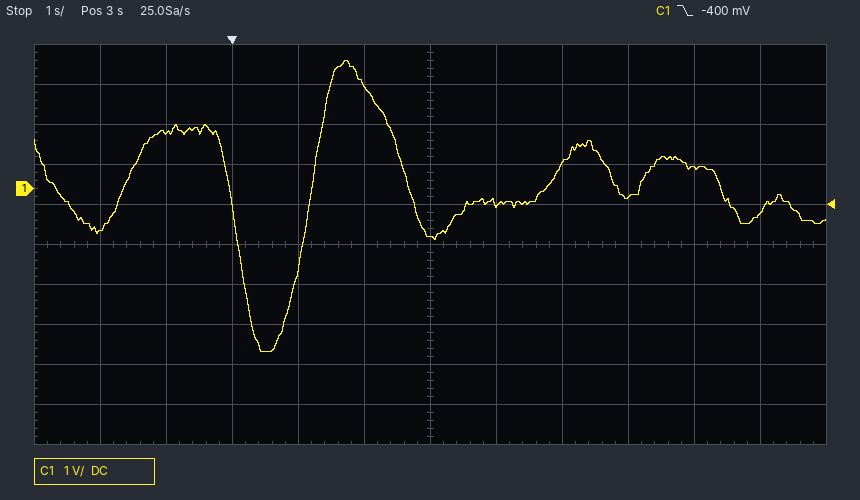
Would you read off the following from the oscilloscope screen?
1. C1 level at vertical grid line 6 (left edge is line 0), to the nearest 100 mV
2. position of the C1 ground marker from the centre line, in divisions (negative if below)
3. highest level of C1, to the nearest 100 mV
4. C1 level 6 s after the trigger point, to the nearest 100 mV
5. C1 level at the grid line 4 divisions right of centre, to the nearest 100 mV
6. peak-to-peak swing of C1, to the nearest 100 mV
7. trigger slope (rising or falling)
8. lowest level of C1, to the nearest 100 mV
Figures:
-1.2 V
+1.4 div
3.2 V
-200 mV
500 mV
7.3 V
falling
-4.1 V
